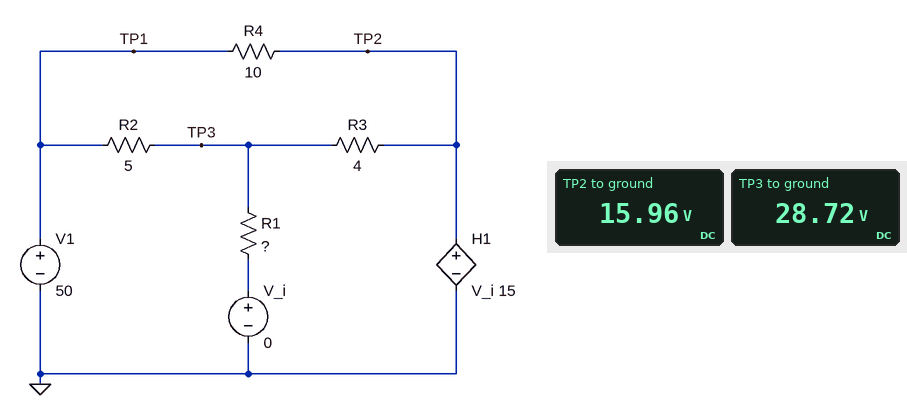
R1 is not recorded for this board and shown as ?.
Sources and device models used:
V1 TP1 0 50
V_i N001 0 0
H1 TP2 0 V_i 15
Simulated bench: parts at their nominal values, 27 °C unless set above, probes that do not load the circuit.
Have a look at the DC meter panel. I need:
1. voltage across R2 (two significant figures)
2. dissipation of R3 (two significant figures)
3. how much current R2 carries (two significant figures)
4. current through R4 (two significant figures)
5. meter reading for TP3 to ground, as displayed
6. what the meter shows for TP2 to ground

21 V
41 W
4.3 A
3.4 A
28.72 V
15.96 V
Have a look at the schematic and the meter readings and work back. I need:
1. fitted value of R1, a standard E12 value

27 Ω
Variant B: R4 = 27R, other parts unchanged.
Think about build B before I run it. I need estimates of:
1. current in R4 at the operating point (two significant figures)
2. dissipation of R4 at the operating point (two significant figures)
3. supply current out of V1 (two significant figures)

1.3 A
43 W
5.5 A
